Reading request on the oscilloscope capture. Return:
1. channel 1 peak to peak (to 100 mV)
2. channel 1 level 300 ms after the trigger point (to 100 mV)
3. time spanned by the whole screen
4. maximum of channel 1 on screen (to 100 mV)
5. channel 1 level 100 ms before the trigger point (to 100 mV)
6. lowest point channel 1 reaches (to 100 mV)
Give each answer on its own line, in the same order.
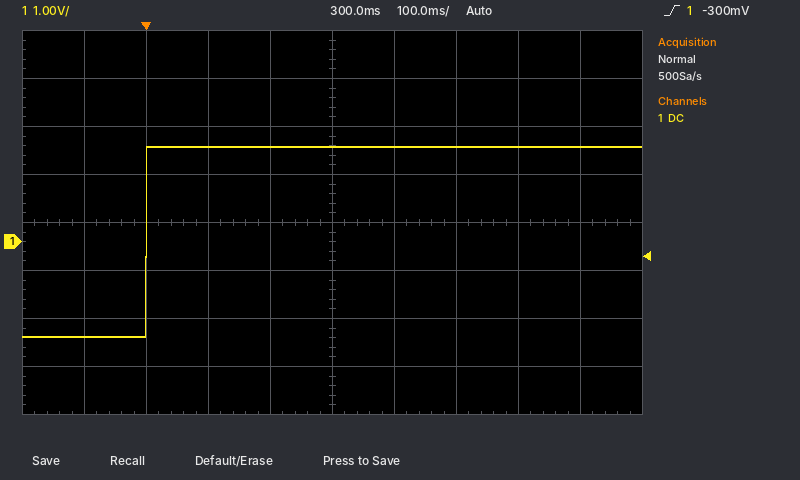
4.0 V
2.0 V
1 s
2.0 V
-2.0 V
-2.0 V
